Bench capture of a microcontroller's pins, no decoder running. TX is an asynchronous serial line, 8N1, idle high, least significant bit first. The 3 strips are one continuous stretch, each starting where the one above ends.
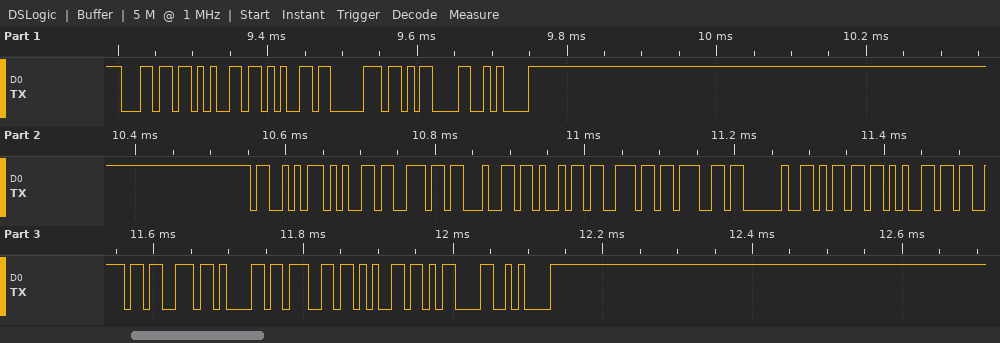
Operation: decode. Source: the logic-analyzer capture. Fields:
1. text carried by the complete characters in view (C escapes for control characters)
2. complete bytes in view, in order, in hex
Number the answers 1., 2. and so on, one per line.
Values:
1. "leep\r\nSending message\r\n"
2. 6C 65 65 70 0D 0A 53 65 6E 64 69 6E 67 20 6D 65 73 73 61 67 65 0D 0A
